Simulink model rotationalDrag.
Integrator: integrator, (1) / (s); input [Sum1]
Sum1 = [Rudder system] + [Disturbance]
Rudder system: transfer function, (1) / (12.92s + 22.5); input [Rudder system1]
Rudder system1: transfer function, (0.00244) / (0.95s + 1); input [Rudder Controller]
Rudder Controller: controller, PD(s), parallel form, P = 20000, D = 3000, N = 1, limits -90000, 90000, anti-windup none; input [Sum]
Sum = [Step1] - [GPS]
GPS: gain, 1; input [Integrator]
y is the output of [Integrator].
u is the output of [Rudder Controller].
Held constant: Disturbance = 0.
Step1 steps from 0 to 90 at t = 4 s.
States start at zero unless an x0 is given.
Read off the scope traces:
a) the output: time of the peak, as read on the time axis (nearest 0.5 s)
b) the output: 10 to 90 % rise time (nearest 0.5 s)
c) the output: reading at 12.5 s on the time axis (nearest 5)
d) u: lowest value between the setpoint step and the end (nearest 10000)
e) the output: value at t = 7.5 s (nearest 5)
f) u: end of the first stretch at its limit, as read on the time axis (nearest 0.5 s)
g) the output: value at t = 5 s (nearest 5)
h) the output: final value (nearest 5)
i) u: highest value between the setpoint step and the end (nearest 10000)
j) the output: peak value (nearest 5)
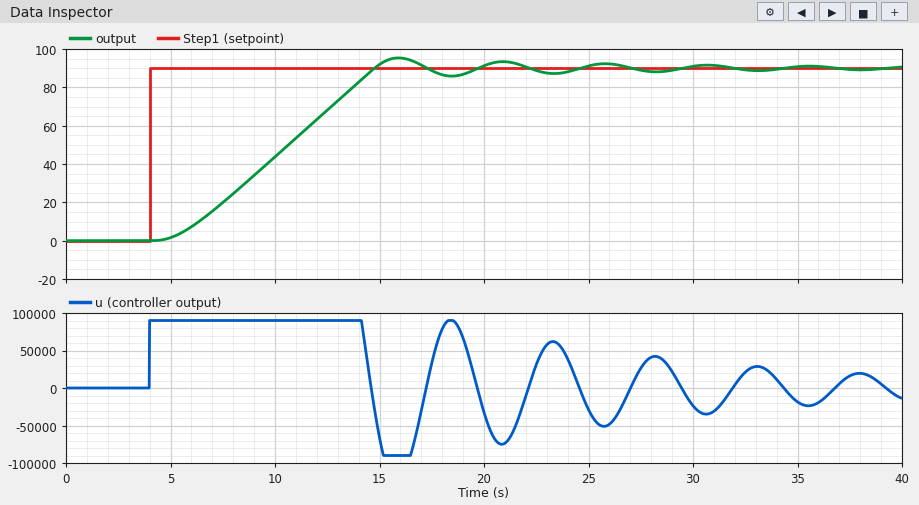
16.0 s
7.5 s
70
-90000
20
14.0 s
0
90
90000
95
